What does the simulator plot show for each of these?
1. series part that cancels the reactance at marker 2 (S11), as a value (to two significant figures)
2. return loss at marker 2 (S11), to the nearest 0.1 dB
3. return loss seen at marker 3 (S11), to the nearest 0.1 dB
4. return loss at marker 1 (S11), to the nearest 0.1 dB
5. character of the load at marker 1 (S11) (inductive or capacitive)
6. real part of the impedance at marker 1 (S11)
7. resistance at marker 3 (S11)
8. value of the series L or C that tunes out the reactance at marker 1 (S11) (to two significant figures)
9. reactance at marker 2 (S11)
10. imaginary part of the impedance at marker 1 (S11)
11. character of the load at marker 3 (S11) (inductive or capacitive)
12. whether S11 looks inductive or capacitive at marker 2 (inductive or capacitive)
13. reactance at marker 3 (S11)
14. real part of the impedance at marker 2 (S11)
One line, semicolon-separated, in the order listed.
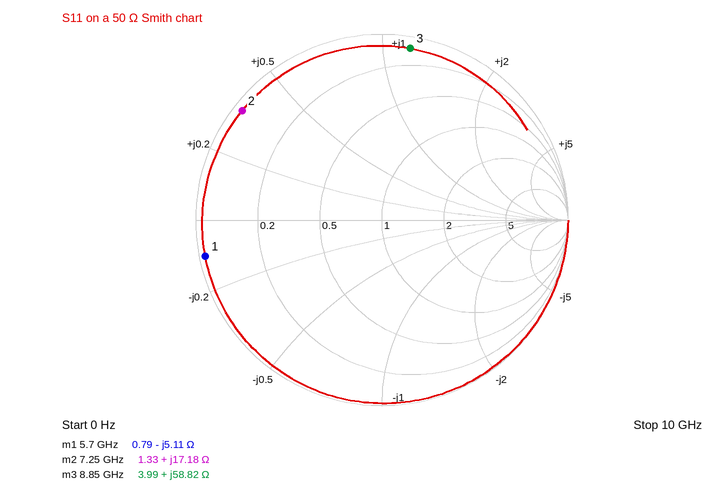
1.3 pF; 0.4 dB; 0.6 dB; 0.3 dB; capacitive; 0.79 Ω; 3.99 Ω; 140 pH; +17.18 Ω; -5.11 Ω; inductive; inductive; +58.82 Ω; 1.33 Ω
